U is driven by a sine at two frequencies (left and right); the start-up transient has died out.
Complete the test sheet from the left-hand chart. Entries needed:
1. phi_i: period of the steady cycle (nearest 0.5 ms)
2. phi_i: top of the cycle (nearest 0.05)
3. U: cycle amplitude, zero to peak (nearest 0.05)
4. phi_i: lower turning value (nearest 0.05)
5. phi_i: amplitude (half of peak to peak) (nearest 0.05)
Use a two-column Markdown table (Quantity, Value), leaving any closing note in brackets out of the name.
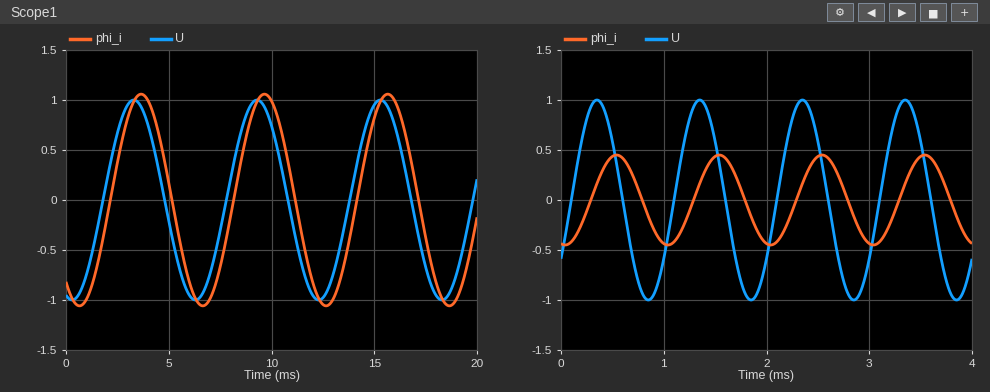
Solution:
| Quantity | Value |
|---|---|
| phi_i: period of the steady cycle | 6.0 ms |
| phi_i: top of the cycle | 1.05 |
| U: cycle amplitude, zero to peak | 1.00 |
| phi_i: lower turning value | -1.05 |
| phi_i: amplitude (half of peak to peak) | 1.05 |
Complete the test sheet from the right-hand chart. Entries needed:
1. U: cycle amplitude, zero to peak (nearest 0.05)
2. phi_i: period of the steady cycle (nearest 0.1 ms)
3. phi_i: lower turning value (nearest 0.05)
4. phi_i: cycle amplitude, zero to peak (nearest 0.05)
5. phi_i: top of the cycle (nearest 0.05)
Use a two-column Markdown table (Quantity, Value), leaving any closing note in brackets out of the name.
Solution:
| Quantity | Value |
|---|---|
| U: cycle amplitude, zero to peak | 1.00 |
| phi_i: period of the steady cycle | 1.0 ms |
| phi_i: lower turning value | -0.45 |
| phi_i: cycle amplitude, zero to peak | 0.45 |
| phi_i: top of the cycle | 0.45 |
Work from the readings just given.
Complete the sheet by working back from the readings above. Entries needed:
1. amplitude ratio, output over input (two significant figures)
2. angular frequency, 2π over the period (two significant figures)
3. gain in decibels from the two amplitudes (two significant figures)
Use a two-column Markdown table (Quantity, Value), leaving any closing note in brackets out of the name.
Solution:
| Quantity | Value |
|---|---|
| amplitude ratio, output over input | 0.45 |
| angular frequency, 2π over the period | 6.3 rad/ms |
| gain in decibels from the two amplitudes | -6.9 dB |
